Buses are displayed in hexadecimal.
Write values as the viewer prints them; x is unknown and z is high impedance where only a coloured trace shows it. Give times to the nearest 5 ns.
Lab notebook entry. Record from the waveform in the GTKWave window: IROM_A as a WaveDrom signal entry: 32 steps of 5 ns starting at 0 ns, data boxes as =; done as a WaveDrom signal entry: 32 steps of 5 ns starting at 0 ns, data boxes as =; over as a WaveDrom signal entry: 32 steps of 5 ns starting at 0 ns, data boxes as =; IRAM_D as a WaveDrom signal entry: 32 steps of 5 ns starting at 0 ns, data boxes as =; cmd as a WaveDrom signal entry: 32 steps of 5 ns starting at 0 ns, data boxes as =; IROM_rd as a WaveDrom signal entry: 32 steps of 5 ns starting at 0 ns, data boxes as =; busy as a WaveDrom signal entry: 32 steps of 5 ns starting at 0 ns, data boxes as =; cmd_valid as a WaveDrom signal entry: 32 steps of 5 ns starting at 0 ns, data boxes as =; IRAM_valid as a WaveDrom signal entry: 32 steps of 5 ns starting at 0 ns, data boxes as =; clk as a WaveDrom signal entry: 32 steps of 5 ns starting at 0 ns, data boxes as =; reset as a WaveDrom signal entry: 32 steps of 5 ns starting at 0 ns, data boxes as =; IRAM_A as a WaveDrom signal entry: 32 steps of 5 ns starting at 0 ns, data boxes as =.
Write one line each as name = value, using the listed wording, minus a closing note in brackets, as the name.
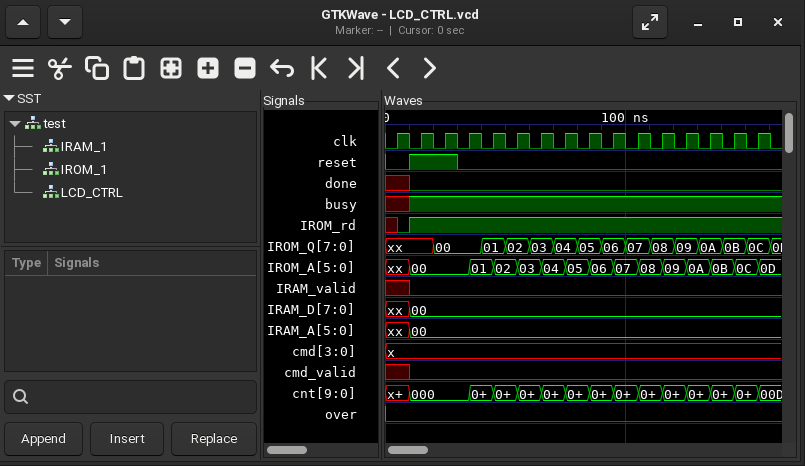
IROM_A as a WaveDrom signal entry: 32 steps of 5 ns starting at 0 ns, data boxes as = = {name: 'IROM_A', wave: 'x.=....=.=.=.=.=.=.=.=.=.=.=.=.=', data: '00 01 02 03 04 05 06 07 08 09 0A 0B 0C 0D'}
done as a WaveDrom signal entry: 32 steps of 5 ns starting at 0 ns, data boxes as = = {name: 'done', wave: 'x.0.............................'}
over as a WaveDrom signal entry: 32 steps of 5 ns starting at 0 ns, data boxes as = = {name: 'over', wave: '0...............................'}
IRAM_D as a WaveDrom signal entry: 32 steps of 5 ns starting at 0 ns, data boxes as = = {name: 'IRAM_D', wave: 'x.=.............................', data: '00'}
cmd as a WaveDrom signal entry: 32 steps of 5 ns starting at 0 ns, data boxes as = = {name: 'cmd', wave: 'x...............................'}
IROM_rd as a WaveDrom signal entry: 32 steps of 5 ns starting at 0 ns, data boxes as = = {name: 'IROM_rd', wave: 'x01.............................'}
busy as a WaveDrom signal entry: 32 steps of 5 ns starting at 0 ns, data boxes as = = {name: 'busy', wave: 'x.1.............................'}
cmd_valid as a WaveDrom signal entry: 32 steps of 5 ns starting at 0 ns, data boxes as = = {name: 'cmd_valid', wave: 'x.0.............................'}
IRAM_valid as a WaveDrom signal entry: 32 steps of 5 ns starting at 0 ns, data boxes as = = {name: 'IRAM_valid', wave: 'x.0.............................'}
clk as a WaveDrom signal entry: 32 steps of 5 ns starting at 0 ns, data boxes as = = {name: 'clk', wave: '01010101010101010101010101010101'}
reset as a WaveDrom signal entry: 32 steps of 5 ns starting at 0 ns, data boxes as = = {name: 'reset', wave: '0.1...0.........................'}
IRAM_A as a WaveDrom signal entry: 32 steps of 5 ns starting at 0 ns, data boxes as = = {name: 'IRAM_A', wave: 'x.=.............................', data: '00'}
